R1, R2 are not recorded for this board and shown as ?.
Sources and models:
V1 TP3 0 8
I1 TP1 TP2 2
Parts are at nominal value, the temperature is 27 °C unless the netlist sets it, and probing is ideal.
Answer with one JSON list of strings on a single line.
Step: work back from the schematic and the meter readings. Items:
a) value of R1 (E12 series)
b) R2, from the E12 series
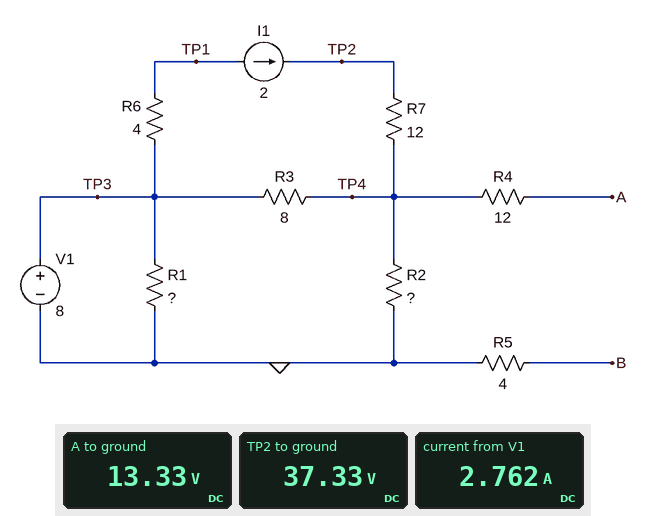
["5.6 Ω", "10 Ω"]
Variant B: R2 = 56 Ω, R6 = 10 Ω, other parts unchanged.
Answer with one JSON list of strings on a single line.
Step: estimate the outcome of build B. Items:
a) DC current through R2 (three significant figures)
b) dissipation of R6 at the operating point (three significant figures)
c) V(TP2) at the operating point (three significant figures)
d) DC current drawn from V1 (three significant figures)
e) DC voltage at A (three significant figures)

["375 mA", "40.0 W", "45.0 V", "1.80 A", "21.0 V"]
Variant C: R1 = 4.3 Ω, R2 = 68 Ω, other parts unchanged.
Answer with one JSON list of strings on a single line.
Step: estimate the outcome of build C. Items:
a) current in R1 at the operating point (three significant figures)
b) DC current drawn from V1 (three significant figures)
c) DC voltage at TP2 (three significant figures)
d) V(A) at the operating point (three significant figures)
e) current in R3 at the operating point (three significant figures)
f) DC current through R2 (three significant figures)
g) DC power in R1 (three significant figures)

["1.86 A", "2.18 A", "45.5 V", "21.5 V", "1.68 A", "316 mA", "14.9 W"]
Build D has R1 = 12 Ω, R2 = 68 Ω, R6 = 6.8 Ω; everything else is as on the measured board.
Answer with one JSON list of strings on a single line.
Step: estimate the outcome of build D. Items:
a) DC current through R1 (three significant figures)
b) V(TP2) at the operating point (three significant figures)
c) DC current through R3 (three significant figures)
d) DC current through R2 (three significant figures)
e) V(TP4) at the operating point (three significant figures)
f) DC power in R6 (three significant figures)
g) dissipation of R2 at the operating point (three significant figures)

["667 mA", "45.5 V", "1.68 A", "316 mA", "21.5 V", "27.2 W", "6.78 W"]
